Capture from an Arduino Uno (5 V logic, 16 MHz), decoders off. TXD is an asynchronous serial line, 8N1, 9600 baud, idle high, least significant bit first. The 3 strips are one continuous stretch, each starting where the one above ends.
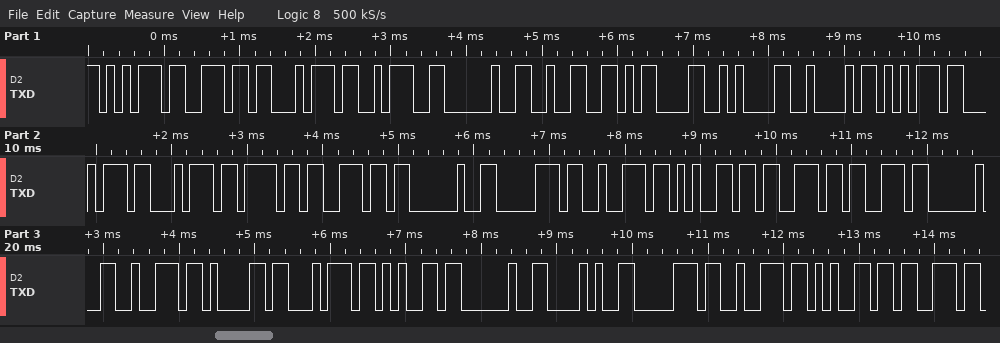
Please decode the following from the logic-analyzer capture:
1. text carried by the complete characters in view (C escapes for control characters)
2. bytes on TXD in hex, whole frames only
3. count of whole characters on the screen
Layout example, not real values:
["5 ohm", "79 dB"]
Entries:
["\"unt: 2\\r\\nButton press rate (pres\"", "75 6E 74 3A 20 32 0D 0A 42 75 74 74 6F 6E 20 70 72 65 73 73 20 72 61 74 65 20 28 70 72 65 73", "31"]
